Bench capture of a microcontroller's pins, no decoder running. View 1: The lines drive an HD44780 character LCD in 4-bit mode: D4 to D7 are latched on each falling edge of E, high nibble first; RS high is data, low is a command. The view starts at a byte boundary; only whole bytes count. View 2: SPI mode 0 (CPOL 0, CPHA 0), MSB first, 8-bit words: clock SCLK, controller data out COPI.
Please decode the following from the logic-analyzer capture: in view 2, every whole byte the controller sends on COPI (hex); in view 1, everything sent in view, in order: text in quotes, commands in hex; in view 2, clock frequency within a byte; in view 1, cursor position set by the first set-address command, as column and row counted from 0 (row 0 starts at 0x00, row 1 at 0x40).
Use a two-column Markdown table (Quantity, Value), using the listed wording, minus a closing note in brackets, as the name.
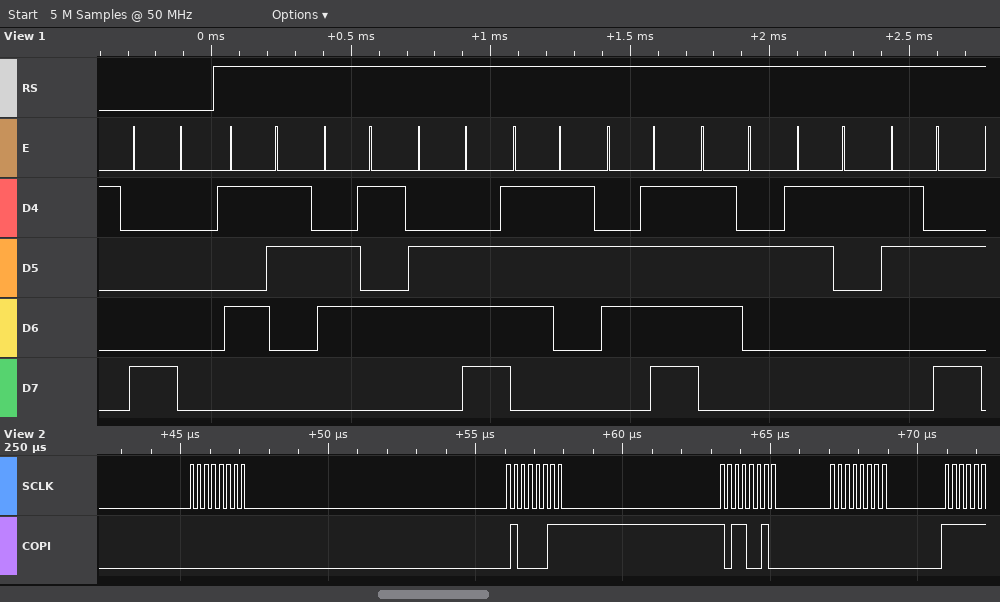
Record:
| Quantity | Value |
|---|---|
| in view 2, every whole byte the controller sends on COPI | 00 43 B2 00 |
| in view 1, everything sent in view, in order: text in quotes, commands in hex | 0x80 "Sensor1:" |
| in view 2, clock frequency within a byte | 4 MHz |
| in view 1, cursor position set by the first set-address command, as column and row counted from 0 | column 0, row 0 |
